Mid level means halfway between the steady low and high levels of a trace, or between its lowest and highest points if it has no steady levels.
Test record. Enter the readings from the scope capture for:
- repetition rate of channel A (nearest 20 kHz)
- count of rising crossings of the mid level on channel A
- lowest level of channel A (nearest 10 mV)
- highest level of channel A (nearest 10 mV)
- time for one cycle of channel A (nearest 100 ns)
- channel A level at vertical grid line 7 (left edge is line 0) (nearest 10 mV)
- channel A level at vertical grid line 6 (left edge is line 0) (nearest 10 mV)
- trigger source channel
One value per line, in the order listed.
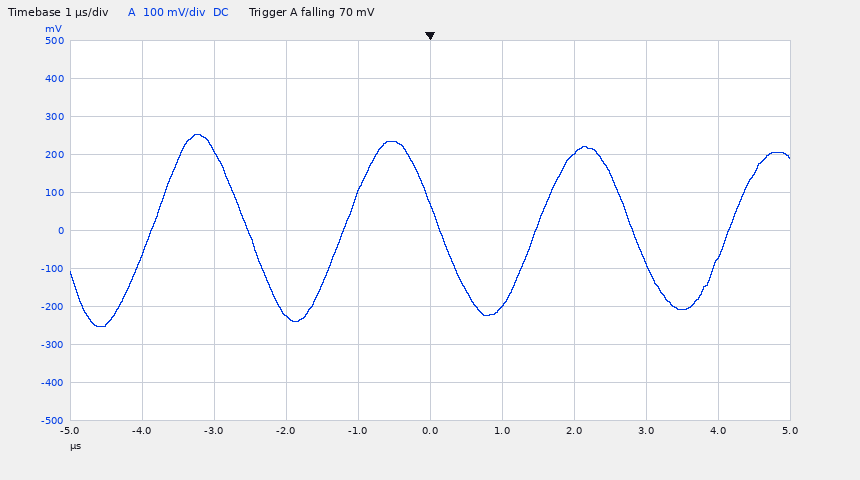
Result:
380 kHz
4
-250 mV
250 mV
2.7 µs
200 mV
-200 mV
channel A
